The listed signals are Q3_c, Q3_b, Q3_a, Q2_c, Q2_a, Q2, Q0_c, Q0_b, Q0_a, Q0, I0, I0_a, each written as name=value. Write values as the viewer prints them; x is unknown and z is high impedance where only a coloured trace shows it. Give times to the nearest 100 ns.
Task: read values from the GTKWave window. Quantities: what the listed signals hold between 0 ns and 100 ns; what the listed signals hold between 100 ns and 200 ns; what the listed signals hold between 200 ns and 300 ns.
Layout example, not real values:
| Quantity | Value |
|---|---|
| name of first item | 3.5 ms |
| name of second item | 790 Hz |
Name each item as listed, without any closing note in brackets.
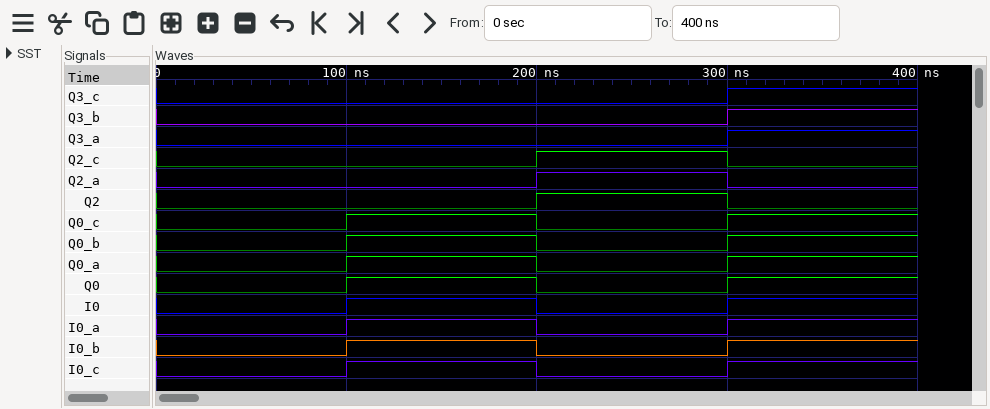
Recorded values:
| Quantity | Value |
|---|---|
| what the listed signals hold between 0 ns and 100 ns | Q3_c=0, Q3_b=0, Q3_a=0, Q2_c=0, Q2_a=0, Q2=0, Q0_c=0, Q0_b=0, Q0_a=0, Q0=0, I0=0, I0_a=0 |
| what the listed signals hold between 100 ns and 200 ns | Q3_c=0, Q3_b=0, Q3_a=0, Q2_c=0, Q2_a=0, Q2=0, Q0_c=1, Q0_b=1, Q0_a=1, Q0=1, I0=1, I0_a=1 |
| what the listed signals hold between 200 ns and 300 ns | Q3_c=0, Q3_b=0, Q3_a=0, Q2_c=1, Q2_a=1, Q2=1, Q0_c=0, Q0_b=0, Q0_a=0, Q0=0, I0=0, I0_a=0 |
